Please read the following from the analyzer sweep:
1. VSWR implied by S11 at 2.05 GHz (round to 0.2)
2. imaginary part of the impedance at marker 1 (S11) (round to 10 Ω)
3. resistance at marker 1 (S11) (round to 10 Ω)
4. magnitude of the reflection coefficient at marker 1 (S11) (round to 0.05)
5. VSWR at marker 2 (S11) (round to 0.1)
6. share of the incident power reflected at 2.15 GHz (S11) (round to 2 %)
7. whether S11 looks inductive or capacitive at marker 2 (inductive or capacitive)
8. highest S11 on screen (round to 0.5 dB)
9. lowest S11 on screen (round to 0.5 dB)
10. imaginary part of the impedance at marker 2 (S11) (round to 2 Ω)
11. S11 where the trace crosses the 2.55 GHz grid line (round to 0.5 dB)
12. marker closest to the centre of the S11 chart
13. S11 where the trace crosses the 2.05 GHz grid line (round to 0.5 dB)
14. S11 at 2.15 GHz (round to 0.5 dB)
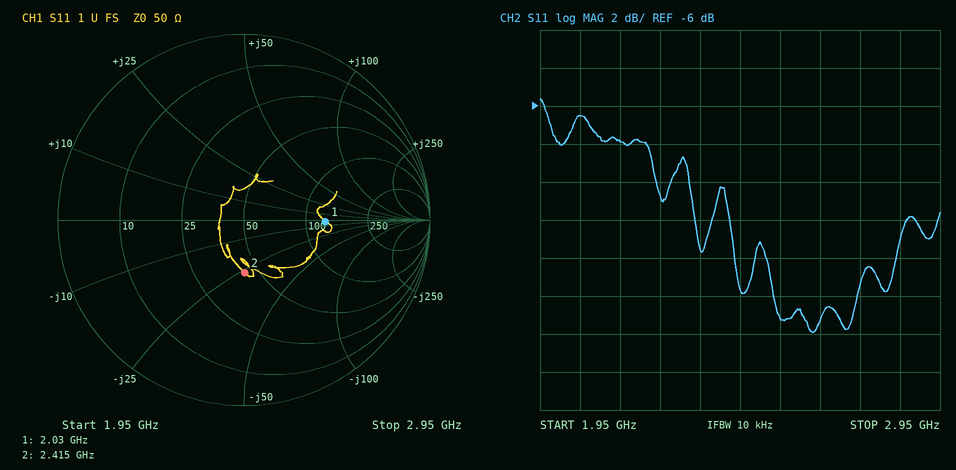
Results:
2.8
0 Ω
130 Ω
0.45
1.8
16 %
capacitive
-5.5 dB
-18.0 dB
-26 Ω
-17.0 dB
marker 2
-6.5 dB
-8.0 dB
